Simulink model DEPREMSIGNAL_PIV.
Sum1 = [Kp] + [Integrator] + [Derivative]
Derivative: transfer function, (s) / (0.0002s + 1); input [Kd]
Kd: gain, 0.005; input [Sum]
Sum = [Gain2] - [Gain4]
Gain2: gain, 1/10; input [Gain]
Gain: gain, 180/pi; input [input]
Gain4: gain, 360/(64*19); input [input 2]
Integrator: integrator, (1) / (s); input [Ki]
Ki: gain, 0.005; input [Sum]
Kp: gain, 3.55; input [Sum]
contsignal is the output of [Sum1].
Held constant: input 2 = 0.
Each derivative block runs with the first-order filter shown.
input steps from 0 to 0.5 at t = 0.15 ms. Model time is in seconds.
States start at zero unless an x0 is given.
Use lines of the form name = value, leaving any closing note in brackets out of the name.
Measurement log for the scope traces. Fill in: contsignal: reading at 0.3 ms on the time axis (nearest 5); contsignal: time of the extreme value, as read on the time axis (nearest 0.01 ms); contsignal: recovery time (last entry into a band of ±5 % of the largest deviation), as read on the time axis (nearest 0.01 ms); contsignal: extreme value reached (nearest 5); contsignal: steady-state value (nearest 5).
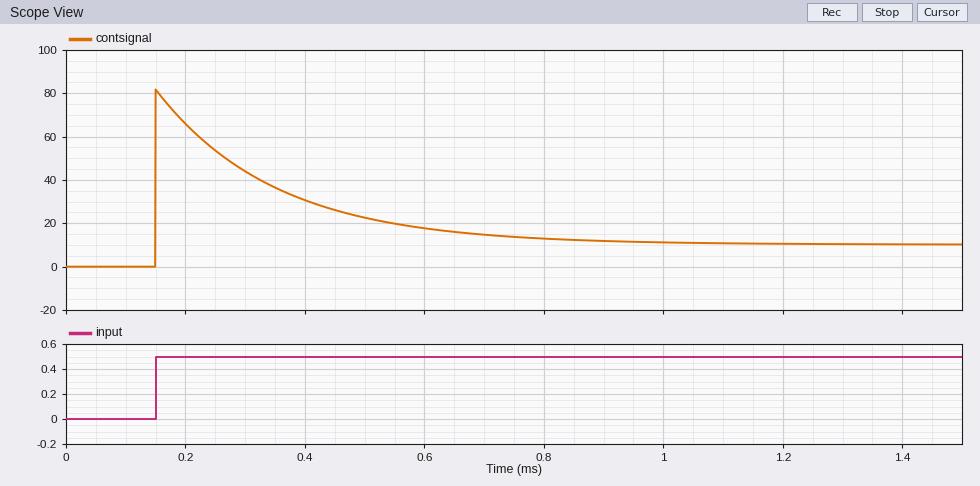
contsignal: reading at 0.3 ms on the time axis = 45
contsignal: time of the extreme value, as read on the time axis = 0.15 ms
contsignal: recovery time (last entry into a band of ±5 % of the largest deviation), as read on the time axis = 0.72 ms
contsignal: extreme value reached = 80
contsignal: steady-state value = 10
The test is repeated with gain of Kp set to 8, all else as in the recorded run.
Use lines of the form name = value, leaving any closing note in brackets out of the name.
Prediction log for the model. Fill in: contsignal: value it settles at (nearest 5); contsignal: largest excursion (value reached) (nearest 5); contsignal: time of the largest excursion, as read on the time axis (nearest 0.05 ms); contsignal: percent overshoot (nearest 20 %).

contsignal: value it settles at = 25
contsignal: largest excursion (value reached) = 95
contsignal: time of the largest excursion, as read on the time axis = 0.15 ms
contsignal: percent overshoot = 320 %
